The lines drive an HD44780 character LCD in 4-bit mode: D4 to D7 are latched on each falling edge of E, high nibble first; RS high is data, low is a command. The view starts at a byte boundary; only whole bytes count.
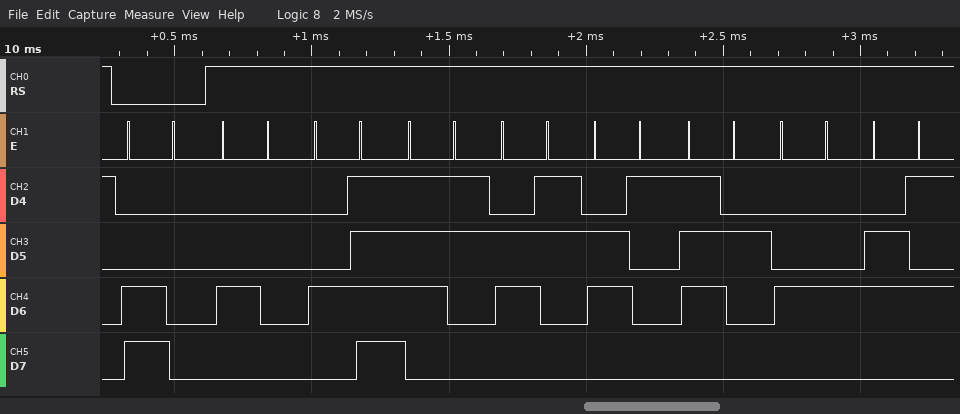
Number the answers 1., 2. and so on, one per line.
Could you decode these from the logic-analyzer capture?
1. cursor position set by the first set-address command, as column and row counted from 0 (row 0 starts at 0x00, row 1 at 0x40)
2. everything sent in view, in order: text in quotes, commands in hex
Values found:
1. column 0, row 1
2. 0xC0 "@OscarDe"
